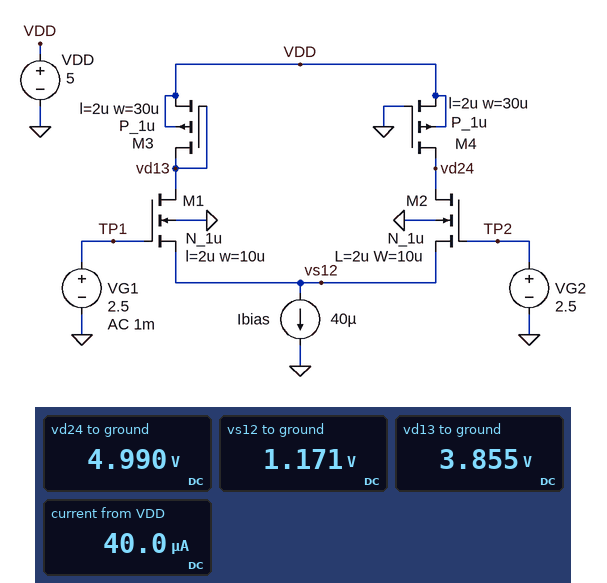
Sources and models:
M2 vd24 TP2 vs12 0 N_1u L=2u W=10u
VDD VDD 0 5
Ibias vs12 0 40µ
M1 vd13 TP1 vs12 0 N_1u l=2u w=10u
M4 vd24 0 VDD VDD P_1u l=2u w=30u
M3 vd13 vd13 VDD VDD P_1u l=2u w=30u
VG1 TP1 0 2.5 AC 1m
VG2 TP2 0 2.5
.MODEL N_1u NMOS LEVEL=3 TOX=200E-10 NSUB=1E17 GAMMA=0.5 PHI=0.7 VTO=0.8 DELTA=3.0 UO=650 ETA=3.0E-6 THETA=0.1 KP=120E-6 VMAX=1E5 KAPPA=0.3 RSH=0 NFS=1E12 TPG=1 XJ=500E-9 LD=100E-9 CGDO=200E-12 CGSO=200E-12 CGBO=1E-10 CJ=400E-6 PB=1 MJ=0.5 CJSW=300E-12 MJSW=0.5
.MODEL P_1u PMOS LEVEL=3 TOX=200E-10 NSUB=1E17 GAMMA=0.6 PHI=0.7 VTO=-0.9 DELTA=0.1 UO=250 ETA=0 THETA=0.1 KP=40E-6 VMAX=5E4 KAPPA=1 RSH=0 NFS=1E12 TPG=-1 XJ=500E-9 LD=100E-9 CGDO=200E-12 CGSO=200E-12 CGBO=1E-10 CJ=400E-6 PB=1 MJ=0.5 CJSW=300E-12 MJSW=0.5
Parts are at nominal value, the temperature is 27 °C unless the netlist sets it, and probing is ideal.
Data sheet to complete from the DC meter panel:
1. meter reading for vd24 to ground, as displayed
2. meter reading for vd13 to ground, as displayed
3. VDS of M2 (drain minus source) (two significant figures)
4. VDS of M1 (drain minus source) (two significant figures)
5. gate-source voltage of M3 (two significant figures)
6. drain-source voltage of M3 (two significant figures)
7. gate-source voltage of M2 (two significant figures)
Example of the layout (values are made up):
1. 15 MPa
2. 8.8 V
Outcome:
1. 4.990 V
2. 3.855 V
3. 3.8 V
4. 2.7 V
5. -1.1 V
6. -1.1 V
7. 1.3 V
